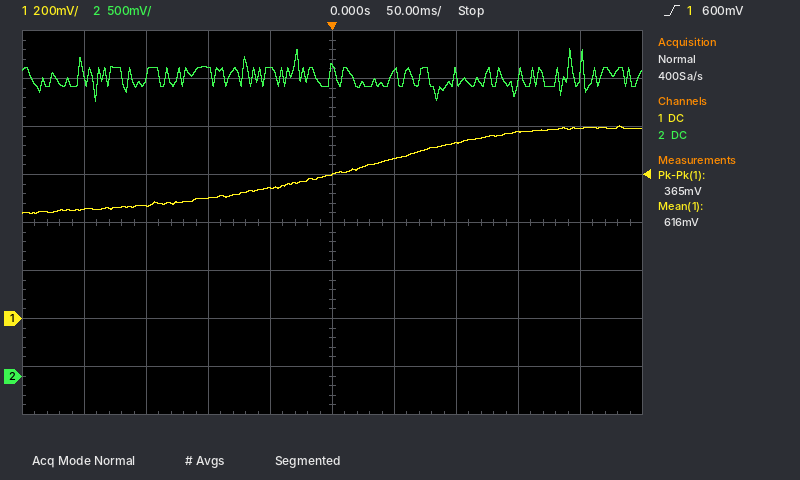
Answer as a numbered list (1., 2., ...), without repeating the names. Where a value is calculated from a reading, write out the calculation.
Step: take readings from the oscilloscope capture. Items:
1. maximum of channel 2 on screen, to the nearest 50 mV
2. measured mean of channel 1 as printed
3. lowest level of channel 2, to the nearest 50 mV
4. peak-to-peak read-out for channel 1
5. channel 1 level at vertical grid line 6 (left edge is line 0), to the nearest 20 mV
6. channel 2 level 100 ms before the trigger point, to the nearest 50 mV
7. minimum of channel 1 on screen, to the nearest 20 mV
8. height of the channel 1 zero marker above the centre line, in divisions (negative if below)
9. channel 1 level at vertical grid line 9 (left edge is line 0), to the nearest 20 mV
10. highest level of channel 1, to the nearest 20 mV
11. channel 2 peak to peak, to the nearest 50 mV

1. 3.40 V
2. 616 mV
3. 2.85 V
4. 365 mV
5. 660 mV
6. 3.20 V
7. 440 mV
8. -2.0 div
9. 800 mV
10. 800 mV
11. 3.40 V − (2.85 V) = 550 mV
